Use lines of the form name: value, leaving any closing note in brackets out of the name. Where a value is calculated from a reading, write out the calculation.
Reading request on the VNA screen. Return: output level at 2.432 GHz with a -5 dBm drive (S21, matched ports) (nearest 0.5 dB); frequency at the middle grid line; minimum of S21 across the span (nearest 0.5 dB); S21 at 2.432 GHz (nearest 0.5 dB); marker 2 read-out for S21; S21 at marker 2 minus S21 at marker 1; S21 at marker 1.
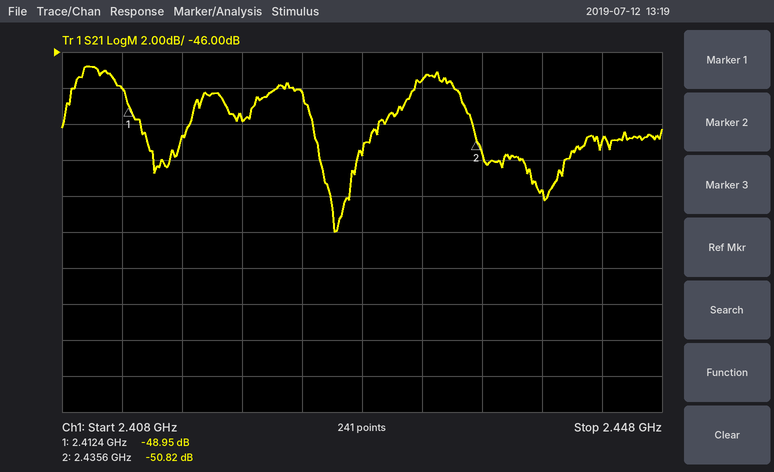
output level at 2.432 GHz with a -5 dBm drive (S21, matched ports): -5 dBm + (-47.5 dB) = -52.5 dBm
frequency at the middle grid line: 2.428 GHz
minimum of S21 across the span: -56.0 dB
S21 at 2.432 GHz: -47.5 dB
marker 2 read-out for S21: -50.82 dB
S21 at marker 2 minus S21 at marker 1: -50.82 − (-48.95) = -1.87 dB
S21 at marker 1: -48.95 dB
